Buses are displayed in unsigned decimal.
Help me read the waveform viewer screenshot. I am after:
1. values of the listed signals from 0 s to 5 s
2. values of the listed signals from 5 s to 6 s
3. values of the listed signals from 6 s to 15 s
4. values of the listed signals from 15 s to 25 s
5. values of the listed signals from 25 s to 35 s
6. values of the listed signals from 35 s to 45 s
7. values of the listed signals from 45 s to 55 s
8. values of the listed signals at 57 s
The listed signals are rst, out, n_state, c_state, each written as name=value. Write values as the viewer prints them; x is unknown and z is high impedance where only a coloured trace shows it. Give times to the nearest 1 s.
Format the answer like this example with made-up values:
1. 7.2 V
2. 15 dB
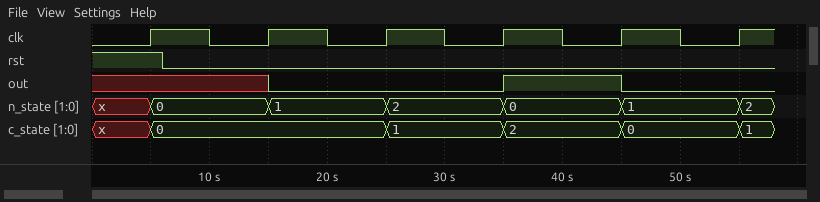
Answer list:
1. rst=1, out=x, n_state=x, c_state=x
2. rst=1, out=x, n_state=0, c_state=0
3. rst=0, out=x, n_state=0, c_state=0
4. rst=0, out=0, n_state=1, c_state=0
5. rst=0, out=0, n_state=2, c_state=1
6. rst=0, out=1, n_state=0, c_state=2
7. rst=0, out=0, n_state=1, c_state=0
8. rst=0, out=0, n_state=2, c_state=1
